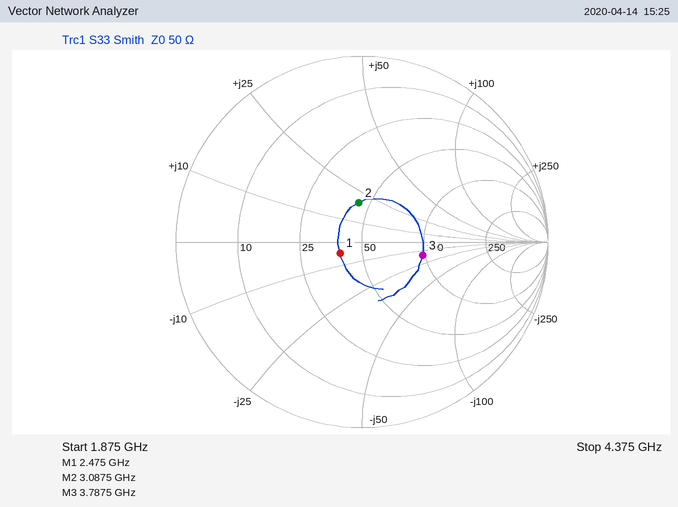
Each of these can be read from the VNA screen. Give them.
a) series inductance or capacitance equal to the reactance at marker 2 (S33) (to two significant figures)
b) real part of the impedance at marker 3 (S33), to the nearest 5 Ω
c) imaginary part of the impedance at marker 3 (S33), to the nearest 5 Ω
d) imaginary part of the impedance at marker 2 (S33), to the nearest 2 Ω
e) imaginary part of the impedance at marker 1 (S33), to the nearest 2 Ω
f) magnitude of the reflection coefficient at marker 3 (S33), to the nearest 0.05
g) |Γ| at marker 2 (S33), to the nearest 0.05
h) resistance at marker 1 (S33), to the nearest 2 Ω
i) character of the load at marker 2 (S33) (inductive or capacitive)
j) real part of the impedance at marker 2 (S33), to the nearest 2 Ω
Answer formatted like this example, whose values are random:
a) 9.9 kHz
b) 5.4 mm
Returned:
a) 1.0 nH
b) 95 Ω
c) -15 Ω
d) +20 Ω
e) -4 Ω
f) 0.35
g) 0.20
h) 40 Ω
i) inductive
j) 44 Ω
